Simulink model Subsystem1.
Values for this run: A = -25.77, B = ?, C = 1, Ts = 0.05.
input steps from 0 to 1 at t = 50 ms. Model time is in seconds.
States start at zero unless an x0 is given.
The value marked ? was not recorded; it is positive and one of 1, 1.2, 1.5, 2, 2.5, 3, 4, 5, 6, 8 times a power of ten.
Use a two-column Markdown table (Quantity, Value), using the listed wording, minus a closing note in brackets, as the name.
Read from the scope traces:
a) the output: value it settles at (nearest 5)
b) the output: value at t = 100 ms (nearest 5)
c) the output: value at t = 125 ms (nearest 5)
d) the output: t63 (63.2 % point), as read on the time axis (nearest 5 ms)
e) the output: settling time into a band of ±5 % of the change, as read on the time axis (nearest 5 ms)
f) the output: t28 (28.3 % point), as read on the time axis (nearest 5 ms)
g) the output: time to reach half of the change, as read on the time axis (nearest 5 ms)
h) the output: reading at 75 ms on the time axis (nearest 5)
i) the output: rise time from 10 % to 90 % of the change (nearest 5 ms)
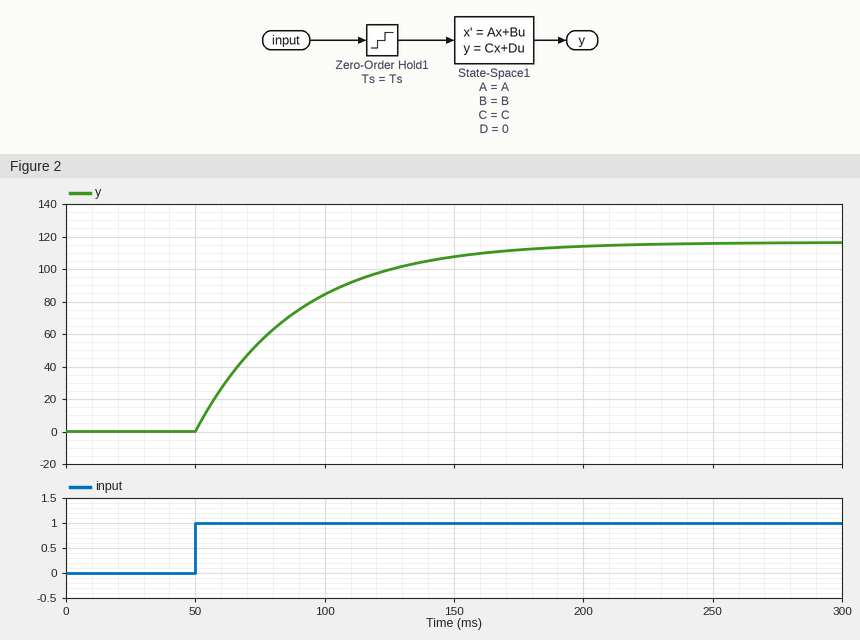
| Quantity | Value |
|---|---|
| the output: value it settles at | 115 |
| the output: value at t = 100 ms | 85 |
| the output: value at t = 125 ms | 100 |
| the output: t63 (63.2 % point), as read on the time axis | 90 ms |
| the output: settling time into a band of ±5 % of the change, as read on the time axis | 165 ms |
| the output: t28 (28.3 % point), as read on the time axis | 65 ms |
| the output: time to reach half of the change, as read on the time axis | 75 ms |
| the output: reading at 75 ms on the time axis | 55 |
| the output: rise time from 10 % to 90 % of the change | 85 ms |
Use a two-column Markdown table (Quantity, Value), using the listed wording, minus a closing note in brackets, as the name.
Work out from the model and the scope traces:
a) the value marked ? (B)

| Quantity | Value |
|---|---|
| the value marked ? | 3000 |
